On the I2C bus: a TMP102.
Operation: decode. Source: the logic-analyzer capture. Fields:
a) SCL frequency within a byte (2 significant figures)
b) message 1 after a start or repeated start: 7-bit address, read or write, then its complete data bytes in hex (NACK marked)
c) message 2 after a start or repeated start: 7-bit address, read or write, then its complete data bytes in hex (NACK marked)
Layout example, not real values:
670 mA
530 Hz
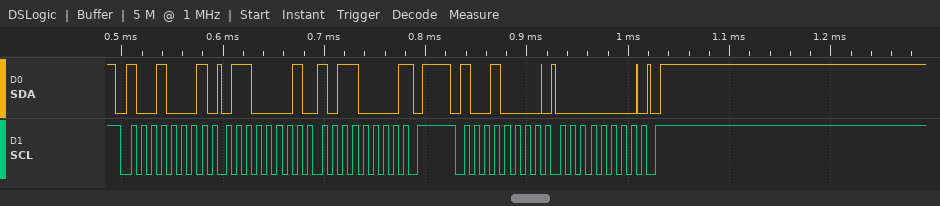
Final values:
100 kHz
0x48 read: 61 B0 NACK
0x48 write: 00
